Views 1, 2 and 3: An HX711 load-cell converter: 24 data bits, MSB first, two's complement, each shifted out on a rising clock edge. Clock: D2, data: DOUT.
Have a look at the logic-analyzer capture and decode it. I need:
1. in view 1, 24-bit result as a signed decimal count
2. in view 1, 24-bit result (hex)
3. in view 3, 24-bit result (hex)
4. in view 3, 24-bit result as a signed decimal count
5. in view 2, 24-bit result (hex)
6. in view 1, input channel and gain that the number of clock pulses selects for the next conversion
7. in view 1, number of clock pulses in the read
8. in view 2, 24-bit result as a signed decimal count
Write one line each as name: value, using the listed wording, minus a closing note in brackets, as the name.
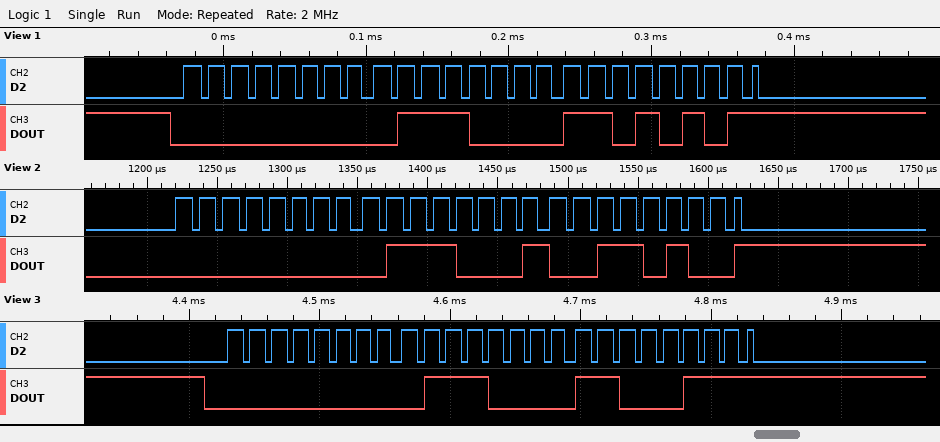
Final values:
in view 1, 24-bit result as a signed decimal count: 28885
in view 1, 24-bit result: 0x0070D5
in view 3, 24-bit result: 0x0070C7
in view 3, 24-bit result as a signed decimal count: 28871
in view 2, 24-bit result: 0x007134
in view 1, input channel and gain that the number of clock pulses selects for the next conversion: channel A, gain 128
in view 1, number of clock pulses in the read: 25
in view 2, 24-bit result as a signed decimal count: 28980
